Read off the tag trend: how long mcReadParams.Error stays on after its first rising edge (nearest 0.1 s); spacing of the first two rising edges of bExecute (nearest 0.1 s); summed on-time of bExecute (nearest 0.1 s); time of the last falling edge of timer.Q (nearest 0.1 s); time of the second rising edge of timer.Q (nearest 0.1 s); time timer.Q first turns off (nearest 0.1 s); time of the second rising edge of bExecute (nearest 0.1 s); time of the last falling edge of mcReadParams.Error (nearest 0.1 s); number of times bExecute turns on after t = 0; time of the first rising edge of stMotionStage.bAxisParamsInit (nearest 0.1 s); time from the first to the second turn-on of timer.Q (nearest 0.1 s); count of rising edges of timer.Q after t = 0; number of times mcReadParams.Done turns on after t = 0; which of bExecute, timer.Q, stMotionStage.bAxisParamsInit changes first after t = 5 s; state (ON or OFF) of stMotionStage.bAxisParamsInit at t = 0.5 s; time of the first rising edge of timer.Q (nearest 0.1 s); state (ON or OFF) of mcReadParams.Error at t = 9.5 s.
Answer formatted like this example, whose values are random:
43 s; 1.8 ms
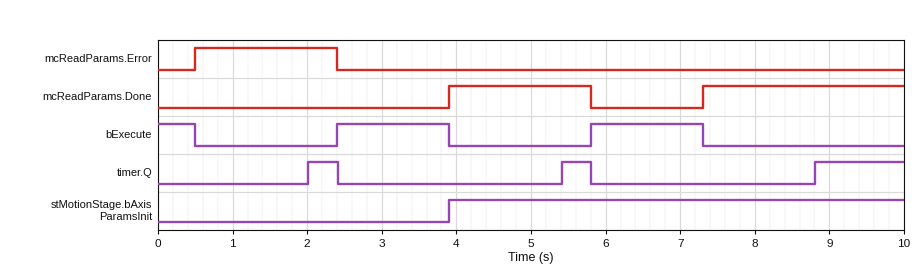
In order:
1.9 s; 3.4 s; 3.5 s; 5.8 s; 5.4 s; 2.4 s; 5.8 s; 2.4 s; 2; 3.9 s; 3.4 s; 3; 2; timer.Q; OFF; 2.0 s; OFF
